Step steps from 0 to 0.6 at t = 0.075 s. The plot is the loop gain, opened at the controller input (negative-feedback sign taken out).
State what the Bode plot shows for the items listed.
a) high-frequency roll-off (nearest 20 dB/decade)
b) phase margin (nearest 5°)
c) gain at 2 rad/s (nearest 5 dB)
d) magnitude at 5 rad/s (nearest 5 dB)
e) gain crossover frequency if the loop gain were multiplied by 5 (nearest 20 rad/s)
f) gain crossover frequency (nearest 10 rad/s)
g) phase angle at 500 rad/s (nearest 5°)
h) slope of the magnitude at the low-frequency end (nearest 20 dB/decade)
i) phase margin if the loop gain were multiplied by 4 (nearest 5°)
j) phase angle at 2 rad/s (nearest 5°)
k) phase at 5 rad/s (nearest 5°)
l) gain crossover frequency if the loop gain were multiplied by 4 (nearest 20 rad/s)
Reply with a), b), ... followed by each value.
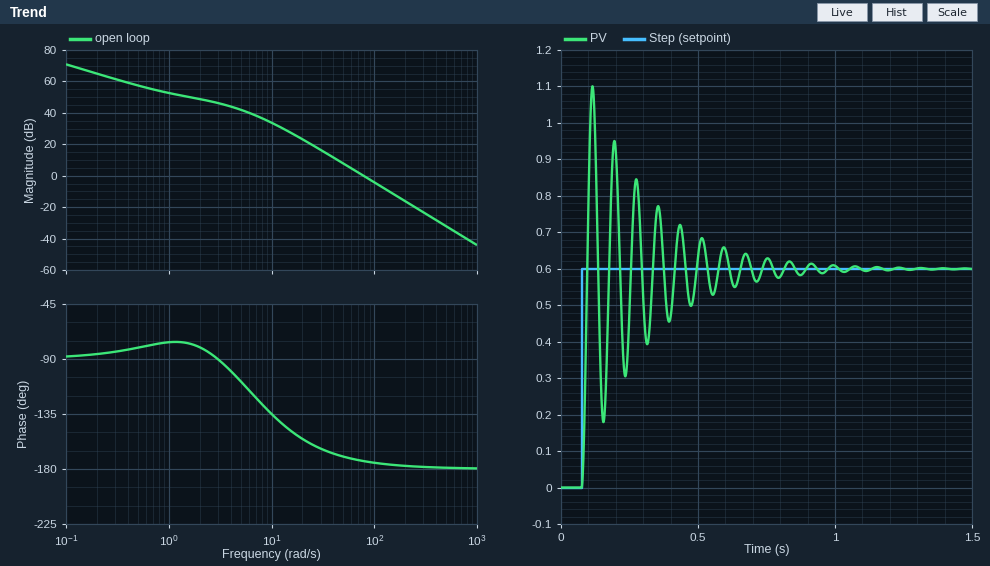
a) -40 dB/decade
b) 5°
c) 50 dB
d) 40 dB
e) 180 rad/s
f) 80 rad/s
g) -180°
h) -20 dB/decade
i) 5°
j) -80°
k) -110°
l) 160 rad/s
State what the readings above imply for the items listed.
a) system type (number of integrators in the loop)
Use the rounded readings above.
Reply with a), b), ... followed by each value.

a) 1
